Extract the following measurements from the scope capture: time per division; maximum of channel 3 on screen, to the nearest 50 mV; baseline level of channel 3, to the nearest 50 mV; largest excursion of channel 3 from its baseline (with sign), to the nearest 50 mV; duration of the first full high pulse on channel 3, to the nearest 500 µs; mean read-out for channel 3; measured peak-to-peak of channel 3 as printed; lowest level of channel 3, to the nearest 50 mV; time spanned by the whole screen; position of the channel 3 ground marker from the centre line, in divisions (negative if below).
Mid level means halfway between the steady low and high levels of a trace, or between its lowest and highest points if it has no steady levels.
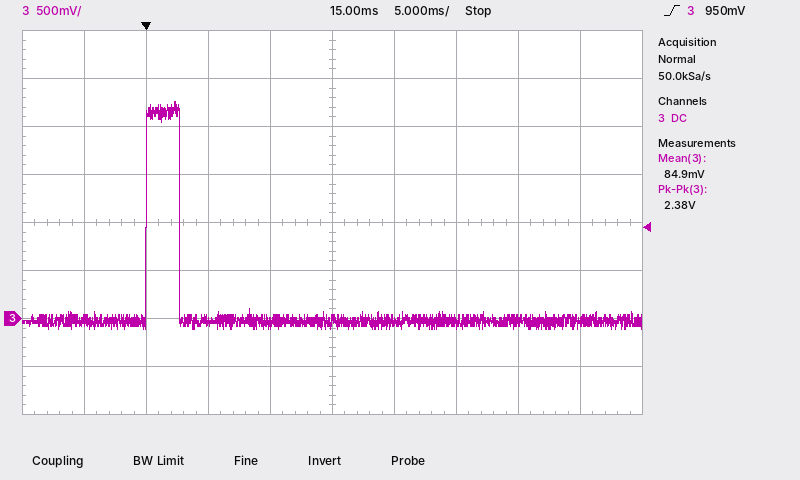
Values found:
5 ms
2.25 V
-50 mV
+2.30 V
2.5 ms
84.9 mV
2.38 V
-100 mV
50 ms
-2.0 div
